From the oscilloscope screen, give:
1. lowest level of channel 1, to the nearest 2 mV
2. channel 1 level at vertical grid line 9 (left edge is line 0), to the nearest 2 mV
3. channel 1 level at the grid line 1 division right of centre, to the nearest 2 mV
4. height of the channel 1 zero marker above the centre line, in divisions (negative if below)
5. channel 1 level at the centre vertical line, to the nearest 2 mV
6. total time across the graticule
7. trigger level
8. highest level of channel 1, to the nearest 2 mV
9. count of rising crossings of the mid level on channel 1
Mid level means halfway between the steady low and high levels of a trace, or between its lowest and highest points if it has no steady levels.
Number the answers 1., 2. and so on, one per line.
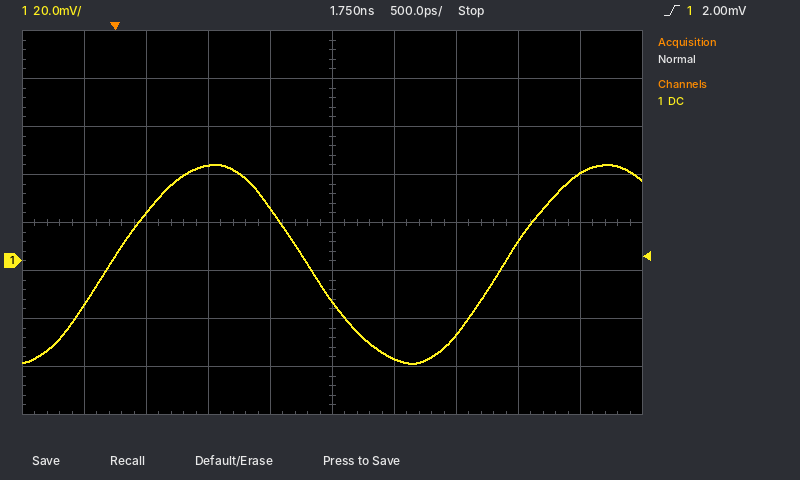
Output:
1. -42 mV
2. 36 mV
3. -40 mV
4. -0.8 div
5. -16 mV
6. 5 ns
7. 2.00 mV
8. 40 mV
9. 2
